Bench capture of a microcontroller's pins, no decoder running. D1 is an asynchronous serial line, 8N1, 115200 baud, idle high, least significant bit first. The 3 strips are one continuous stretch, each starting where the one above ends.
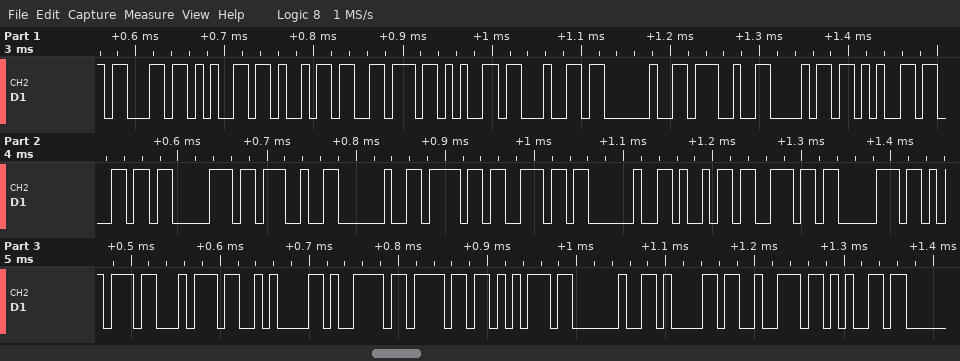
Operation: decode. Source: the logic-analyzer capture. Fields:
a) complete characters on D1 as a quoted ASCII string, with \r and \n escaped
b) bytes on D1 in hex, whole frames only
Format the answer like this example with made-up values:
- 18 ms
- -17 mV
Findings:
- "ceived 'help' on input\nyou are"
- 63 65 69 76 65 64 20 27 68 65 6C 70 27 20 6F 6E 20 69 6E 70 75 74 0A 79 6F 75 20 61 72 65
